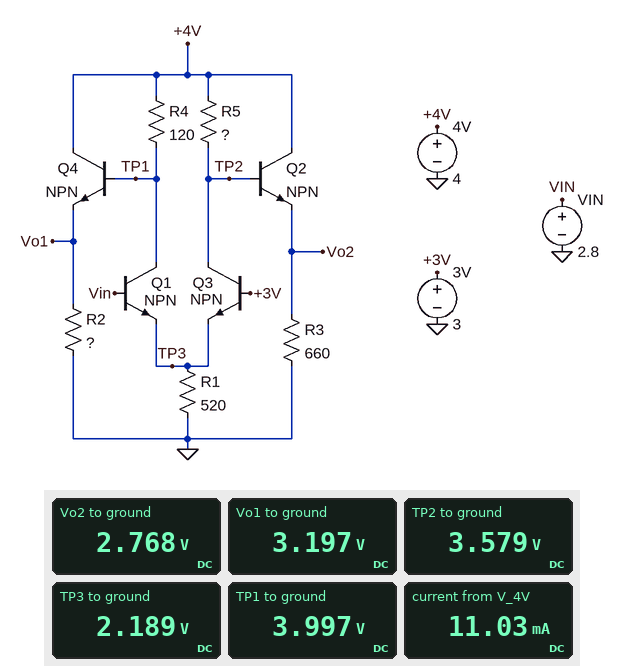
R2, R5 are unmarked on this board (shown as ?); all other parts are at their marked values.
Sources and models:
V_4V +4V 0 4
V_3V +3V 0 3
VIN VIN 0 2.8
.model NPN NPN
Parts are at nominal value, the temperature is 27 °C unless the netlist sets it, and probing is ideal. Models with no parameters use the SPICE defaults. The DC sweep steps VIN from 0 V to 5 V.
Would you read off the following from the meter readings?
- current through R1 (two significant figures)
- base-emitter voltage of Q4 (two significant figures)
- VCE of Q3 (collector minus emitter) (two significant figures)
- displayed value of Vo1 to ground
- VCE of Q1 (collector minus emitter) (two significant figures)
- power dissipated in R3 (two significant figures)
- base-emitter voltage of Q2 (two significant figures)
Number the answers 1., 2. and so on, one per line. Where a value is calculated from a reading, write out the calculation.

1. (2.189 V) / 520 Ω = 4.2 mA
2. 3.997 V - 3.197 V = 800 mV
3. 3.579 V - 2.189 V = 1.4 V
4. 3.197 V
5. 3.997 V - 2.189 V = 1.8 V
6. (2.768 V)^2 / 660 Ω = 12 mW
7. 3.579 V - 2.768 V = 810 mV
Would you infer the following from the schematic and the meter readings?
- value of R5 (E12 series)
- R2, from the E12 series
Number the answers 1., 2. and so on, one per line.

1. 100 Ω
2. 1.2 kΩ
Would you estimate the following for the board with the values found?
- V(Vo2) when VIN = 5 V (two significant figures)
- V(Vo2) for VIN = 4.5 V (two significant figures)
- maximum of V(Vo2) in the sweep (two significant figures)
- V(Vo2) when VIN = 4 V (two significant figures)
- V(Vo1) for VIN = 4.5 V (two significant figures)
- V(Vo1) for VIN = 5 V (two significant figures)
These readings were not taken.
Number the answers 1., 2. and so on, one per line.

1. 3.2 V
2. 3.2 V
3. 3.2 V
4. 3.2 V
5. 2.9 V
6. 3.4 V
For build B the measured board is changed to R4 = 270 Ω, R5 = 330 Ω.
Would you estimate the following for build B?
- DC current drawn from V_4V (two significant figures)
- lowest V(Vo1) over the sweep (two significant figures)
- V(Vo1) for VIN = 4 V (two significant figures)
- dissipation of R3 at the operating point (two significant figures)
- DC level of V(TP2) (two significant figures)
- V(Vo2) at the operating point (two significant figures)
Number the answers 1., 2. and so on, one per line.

1. 9.6 mA
2. 1.9 V
3. 2.4 V
4. 5.0 mW
5. 2.6 V
6. 1.8 V
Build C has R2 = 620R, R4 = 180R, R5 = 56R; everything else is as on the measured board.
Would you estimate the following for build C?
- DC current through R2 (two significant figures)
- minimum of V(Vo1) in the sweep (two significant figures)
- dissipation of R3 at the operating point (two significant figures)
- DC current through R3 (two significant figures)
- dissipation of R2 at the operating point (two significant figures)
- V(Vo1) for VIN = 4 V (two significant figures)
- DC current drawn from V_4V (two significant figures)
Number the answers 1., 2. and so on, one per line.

1. 5.1 mA
2. 2.2 V
3. 13 mW
4. 4.5 mA
5. 16 mW
6. 2.4 V
7. 14 mA
